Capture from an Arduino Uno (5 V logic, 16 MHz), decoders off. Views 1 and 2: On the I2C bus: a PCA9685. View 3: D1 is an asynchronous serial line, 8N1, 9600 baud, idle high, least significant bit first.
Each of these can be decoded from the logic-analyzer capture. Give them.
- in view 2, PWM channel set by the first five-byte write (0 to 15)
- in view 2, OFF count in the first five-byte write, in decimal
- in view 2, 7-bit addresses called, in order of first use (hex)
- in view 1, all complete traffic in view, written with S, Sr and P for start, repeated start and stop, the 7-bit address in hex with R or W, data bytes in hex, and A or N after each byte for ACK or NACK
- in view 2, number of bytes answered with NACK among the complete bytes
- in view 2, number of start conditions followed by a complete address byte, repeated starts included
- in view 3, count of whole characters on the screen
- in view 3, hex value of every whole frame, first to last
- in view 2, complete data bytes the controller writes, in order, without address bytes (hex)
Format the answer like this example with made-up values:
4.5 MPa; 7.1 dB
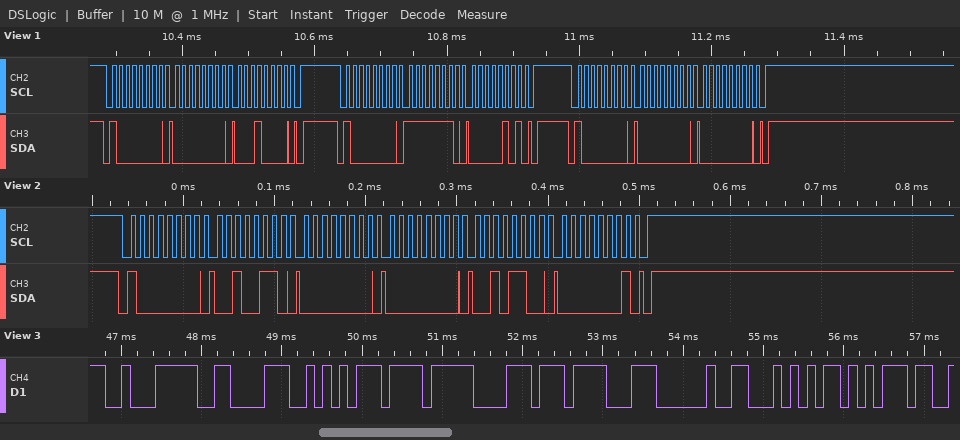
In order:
8; 300; 0x40; S 40W A 00 A 10 A P S 40W A FE A 05 A P S 40W A 00 A 00 A P; 0; 1; 9; E2 86 AA EF B8 8F 20 54 75; 26 00 00 2C 01
